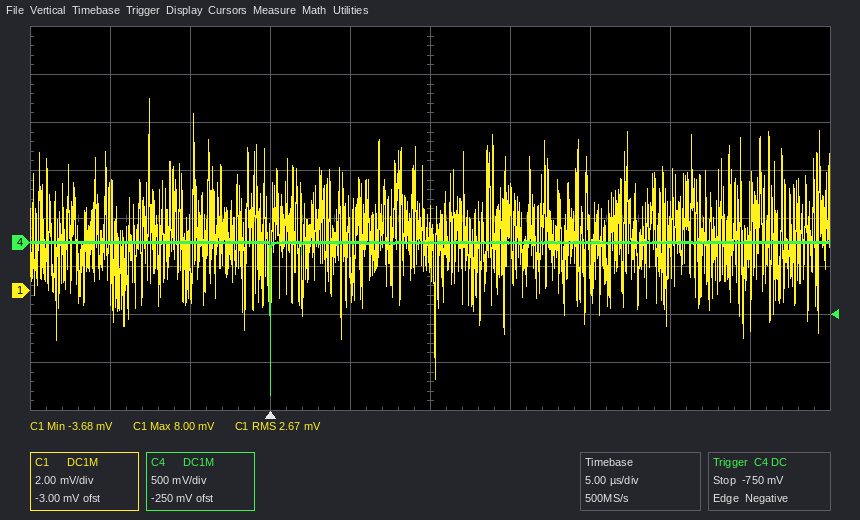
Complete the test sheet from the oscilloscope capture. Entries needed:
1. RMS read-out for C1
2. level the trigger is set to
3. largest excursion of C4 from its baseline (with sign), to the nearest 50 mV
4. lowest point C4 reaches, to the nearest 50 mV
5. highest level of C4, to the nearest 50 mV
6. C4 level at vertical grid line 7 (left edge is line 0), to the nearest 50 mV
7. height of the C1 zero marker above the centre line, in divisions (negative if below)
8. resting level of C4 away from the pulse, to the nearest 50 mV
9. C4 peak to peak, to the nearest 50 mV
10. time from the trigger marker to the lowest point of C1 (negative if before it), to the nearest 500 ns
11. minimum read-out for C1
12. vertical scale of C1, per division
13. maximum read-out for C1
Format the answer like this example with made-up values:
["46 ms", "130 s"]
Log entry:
["2.67 mV", "-750 mV", "-1.60 V", "-1.60 V", "0 mV", "0 mV", "-1.5 div", "0 mV", "1.60 V", "+10.5 µs", "-3.68 mV", "2 mV", "8.00 mV"]
